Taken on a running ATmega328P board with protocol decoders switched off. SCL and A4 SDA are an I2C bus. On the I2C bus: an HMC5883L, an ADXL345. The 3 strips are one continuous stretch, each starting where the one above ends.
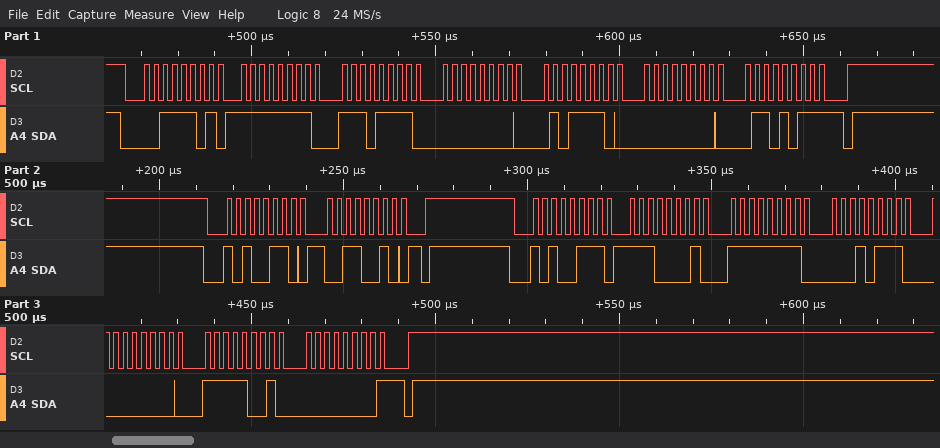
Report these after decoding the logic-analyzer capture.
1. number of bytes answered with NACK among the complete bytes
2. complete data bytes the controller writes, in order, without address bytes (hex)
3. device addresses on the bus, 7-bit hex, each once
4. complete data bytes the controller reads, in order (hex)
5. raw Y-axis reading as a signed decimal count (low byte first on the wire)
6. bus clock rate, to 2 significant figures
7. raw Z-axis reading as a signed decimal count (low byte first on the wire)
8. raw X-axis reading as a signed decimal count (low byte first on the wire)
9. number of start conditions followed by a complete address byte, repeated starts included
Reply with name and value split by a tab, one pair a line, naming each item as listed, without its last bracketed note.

number of bytes answered with NACK among the complete bytes	2
complete data bytes the controller writes, in order, without address bytes	32
device addresses on the bus, 7-bit hex, each once	0x1E 0x53
complete data bytes the controller reads, in order	FF EF 00 5E 00 6B E1 FF 17 00 F9 00
raw Y-axis reading as a signed decimal count	23
bus clock rate, to 2 significant figures	400 kHz
raw Z-axis reading as a signed decimal count	249
raw X-axis reading as a signed decimal count	-31
number of start conditions followed by a complete address byte, repeated starts included	3
